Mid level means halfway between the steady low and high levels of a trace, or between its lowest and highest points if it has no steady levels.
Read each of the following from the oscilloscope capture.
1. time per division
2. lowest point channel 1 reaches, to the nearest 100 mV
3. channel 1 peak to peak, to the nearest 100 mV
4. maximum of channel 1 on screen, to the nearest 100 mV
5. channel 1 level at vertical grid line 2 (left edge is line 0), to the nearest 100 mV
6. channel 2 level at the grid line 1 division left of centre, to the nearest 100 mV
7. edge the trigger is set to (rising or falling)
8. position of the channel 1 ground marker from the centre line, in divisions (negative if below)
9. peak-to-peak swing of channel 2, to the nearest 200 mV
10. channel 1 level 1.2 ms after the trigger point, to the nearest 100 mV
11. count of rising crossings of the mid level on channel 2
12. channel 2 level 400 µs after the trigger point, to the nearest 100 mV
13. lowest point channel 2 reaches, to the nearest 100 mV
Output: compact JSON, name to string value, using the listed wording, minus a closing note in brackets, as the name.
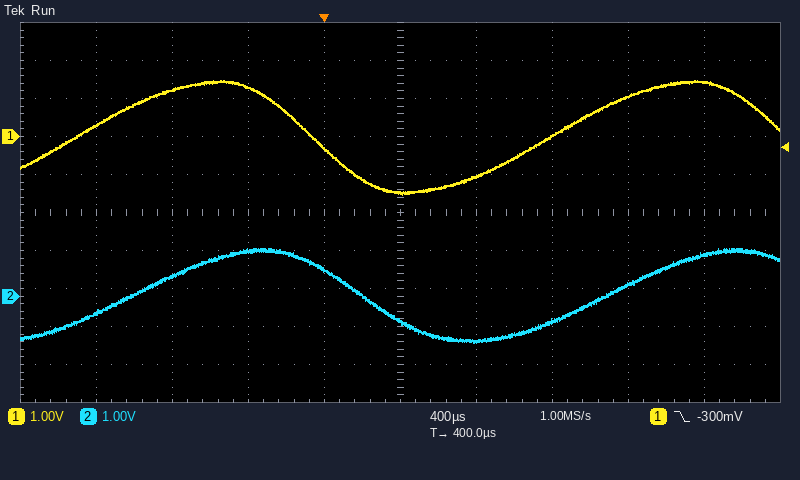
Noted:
{"time per division": "400 µs", "lowest point channel 1 reaches, to the nearest 100 mV": "-1.5 V", "channel 1 peak to peak, to the nearest 100 mV": "3.0 V", "maximum of channel 1 on screen, to the nearest 100 mV": "1.5 V", "channel 1 level at vertical grid line 2 (left edge is line 0), to the nearest 100 mV": "1.2 V", "channel 2 level at the grid line 1 division left of centre, to the nearest 100 mV": "700 mV", "edge the trigger is set to": "falling", "position of the channel 1 ground marker from the centre line, in divisions": "+2.0 div", "peak-to-peak swing of channel 2, to the nearest 200 mV": "2.4 V", "channel 1 level 1.2 ms after the trigger point, to the nearest 100 mV": "0.0 V", "count of rising crossings of the mid level on channel 2": "2", "channel 2 level 400 µs after the trigger point, to the nearest 100 mV": "-700 mV", "lowest point channel 2 reaches, to the nearest 100 mV": "-1.2 V"}
